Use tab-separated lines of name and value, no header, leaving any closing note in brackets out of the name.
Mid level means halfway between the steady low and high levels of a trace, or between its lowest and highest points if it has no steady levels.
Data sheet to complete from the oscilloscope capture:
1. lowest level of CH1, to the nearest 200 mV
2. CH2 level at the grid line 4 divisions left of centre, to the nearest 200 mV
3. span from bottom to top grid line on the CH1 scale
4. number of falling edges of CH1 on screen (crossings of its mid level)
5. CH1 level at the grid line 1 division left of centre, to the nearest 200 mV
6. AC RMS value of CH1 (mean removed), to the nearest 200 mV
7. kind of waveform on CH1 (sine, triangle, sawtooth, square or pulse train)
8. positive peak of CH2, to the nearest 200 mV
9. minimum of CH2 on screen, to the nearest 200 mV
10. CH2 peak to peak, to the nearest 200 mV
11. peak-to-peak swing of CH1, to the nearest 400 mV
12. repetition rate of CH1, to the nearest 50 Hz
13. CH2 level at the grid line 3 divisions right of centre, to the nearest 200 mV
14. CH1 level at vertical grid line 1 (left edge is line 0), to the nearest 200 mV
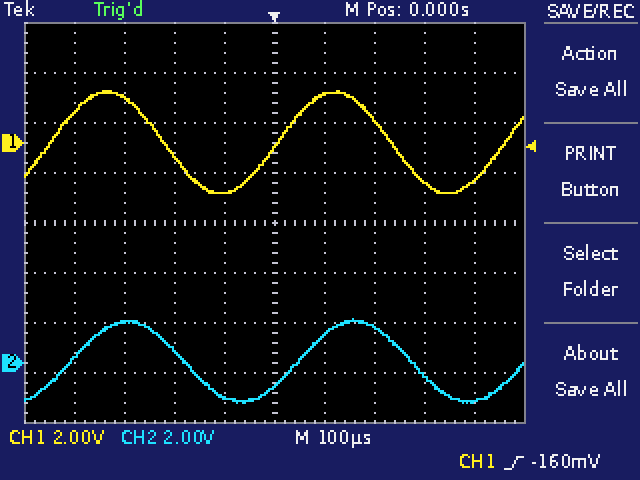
lowest level of CH1, to the nearest 200 mV	-2.0 V
CH2 level at the grid line 4 divisions left of centre, to the nearest 200 mV	200 mV
span from bottom to top grid line on the CH1 scale	16 V
number of falling edges of CH1 on screen	2
CH1 level at the grid line 1 division left of centre, to the nearest 200 mV	-2.0 V
AC RMS value of CH1 (mean removed), to the nearest 200 mV	1.4 V
kind of waveform on CH1	sine
positive peak of CH2, to the nearest 200 mV	1.8 V
minimum of CH2 on screen, to the nearest 200 mV	-1.6 V
CH2 peak to peak, to the nearest 200 mV	3.4 V
peak-to-peak swing of CH1, to the nearest 400 mV	4.0 V
repetition rate of CH1, to the nearest 50 Hz	2.20 kHz
CH2 level at the grid line 3 divisions right of centre, to the nearest 200 mV	-600 mV
CH1 level at vertical grid line 1 (left edge is line 0), to the nearest 200 mV	1.2 V
